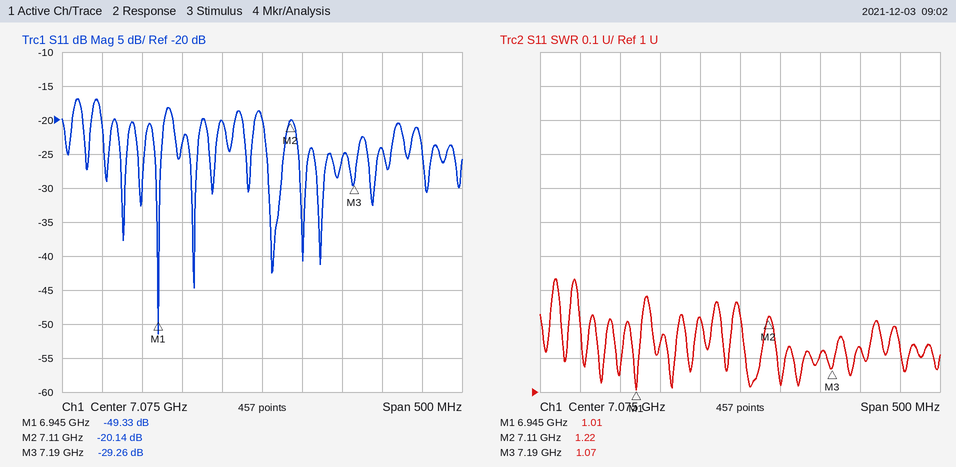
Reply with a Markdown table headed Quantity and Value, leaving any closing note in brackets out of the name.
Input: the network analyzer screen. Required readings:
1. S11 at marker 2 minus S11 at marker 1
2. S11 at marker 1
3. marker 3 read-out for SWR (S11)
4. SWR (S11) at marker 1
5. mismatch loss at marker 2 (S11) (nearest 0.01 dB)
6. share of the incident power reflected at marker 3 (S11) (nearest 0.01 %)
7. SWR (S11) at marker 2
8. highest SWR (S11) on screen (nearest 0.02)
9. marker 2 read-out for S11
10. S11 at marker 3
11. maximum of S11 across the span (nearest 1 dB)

| Quantity | Value |
|---|---|
| S11 at marker 2 minus S11 at marker 1 | 29.19 dB |
| S11 at marker 1 | -49.33 dB |
| marker 3 read-out for SWR | 1.07 |
| SWR (S11) at marker 1 | 1.01 |
| mismatch loss at marker 2 (S11) | 0.04 dB |
| share of the incident power reflected at marker 3 (S11) | 0.12 % |
| SWR (S11) at marker 2 | 1.22 |
| highest SWR (S11) on screen | 1.34 |
| marker 2 read-out for S11 | -20.14 dB |
| S11 at marker 3 | -29.26 dB |
| maximum of S11 across the span | -17 dB |
